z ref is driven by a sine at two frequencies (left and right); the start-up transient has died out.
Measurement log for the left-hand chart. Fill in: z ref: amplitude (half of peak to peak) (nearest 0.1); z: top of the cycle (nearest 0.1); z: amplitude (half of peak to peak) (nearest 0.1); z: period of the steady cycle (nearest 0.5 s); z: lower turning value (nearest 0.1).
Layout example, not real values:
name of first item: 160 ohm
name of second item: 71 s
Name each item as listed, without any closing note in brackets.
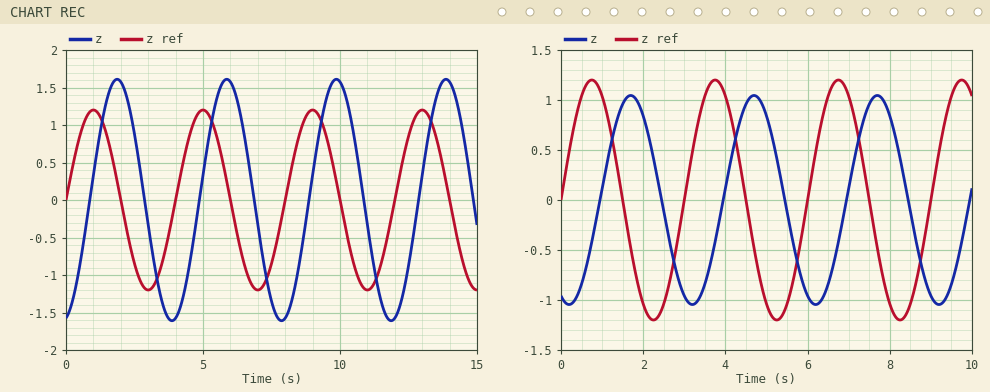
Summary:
z ref: amplitude (half of peak to peak): 1.2
z: top of the cycle: 1.6
z: amplitude (half of peak to peak): 1.6
z: period of the steady cycle: 4.0 s
z: lower turning value: -1.6
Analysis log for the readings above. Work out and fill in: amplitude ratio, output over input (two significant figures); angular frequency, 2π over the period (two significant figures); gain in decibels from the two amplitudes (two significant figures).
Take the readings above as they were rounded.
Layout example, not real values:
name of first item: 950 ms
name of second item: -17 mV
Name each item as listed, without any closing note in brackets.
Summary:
amplitude ratio, output over input: 1.3
angular frequency, 2π over the period: 1.6 rad/s
gain in decibels from the two amplitudes: 2.5 dB
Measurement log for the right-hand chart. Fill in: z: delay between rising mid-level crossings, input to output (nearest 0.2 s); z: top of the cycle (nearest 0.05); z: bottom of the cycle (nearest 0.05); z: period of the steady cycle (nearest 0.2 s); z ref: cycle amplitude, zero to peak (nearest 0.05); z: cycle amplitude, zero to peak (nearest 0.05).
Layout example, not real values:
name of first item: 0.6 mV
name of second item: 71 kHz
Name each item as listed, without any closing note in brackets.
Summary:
z: delay between rising mid-level crossings, input to output: 1.0 s
z: top of the cycle: 1.05
z: bottom of the cycle: -1.05
z: period of the steady cycle: 3.0 s
z ref: cycle amplitude, zero to peak: 1.20
z: cycle amplitude, zero to peak: 1.05
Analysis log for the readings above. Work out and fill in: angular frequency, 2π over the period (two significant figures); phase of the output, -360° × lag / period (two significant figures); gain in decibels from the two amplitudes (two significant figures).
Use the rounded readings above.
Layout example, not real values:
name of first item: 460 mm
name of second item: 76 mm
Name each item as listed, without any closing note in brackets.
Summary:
angular frequency, 2π over the period: 2.1 rad/s
phase of the output, -360° × lag / period: -120°
gain in decibels from the two amplitudes: -1.2 dB
